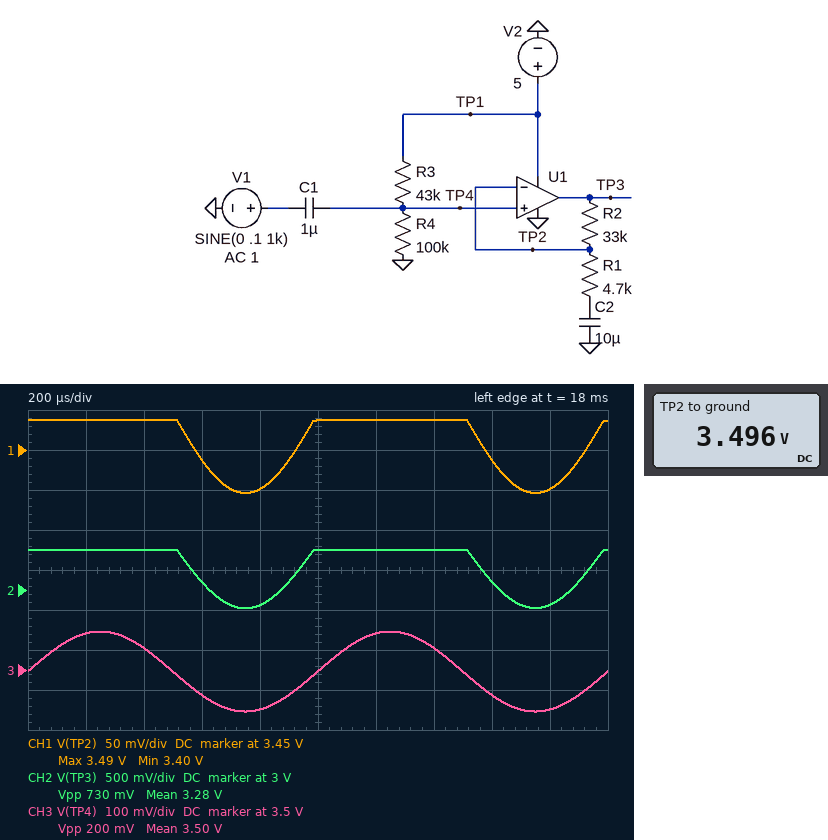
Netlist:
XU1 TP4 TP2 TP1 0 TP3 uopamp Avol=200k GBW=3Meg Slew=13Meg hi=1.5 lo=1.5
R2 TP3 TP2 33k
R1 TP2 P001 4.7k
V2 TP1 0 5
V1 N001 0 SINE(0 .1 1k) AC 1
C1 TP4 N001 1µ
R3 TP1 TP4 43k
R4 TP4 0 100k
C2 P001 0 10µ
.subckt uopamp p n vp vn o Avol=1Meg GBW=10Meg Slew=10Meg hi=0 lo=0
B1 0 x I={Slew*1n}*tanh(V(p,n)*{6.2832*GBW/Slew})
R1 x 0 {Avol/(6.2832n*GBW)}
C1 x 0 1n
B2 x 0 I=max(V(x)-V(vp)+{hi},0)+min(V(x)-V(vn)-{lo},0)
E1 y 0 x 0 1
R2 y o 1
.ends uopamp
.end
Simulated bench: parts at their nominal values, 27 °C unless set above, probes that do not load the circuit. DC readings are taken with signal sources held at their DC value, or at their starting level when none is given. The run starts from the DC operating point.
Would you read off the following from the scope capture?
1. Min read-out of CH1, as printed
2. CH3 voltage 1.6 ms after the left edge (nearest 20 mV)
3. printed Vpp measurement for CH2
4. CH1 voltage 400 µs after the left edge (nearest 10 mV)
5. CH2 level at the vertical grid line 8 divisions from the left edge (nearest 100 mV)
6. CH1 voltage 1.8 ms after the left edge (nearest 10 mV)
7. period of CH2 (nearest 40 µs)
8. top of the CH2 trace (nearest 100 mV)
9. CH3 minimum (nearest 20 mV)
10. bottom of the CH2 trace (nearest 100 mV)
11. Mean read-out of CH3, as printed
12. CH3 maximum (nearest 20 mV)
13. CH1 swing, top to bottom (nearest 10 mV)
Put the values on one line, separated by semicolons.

3.40 V; 3.44 V; 730 mV; 3.49 V; 3.1 V; 3.40 V; 1.00 ms; 3.5 V; 3.40 V; 2.8 V; 3.50 V; 3.60 V; 90 mV
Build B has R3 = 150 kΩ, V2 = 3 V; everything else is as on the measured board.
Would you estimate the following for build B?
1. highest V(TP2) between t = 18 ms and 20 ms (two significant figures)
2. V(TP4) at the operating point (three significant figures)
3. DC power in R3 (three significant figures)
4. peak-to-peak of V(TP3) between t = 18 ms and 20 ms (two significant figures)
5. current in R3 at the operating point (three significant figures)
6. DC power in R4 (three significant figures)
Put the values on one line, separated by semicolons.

1.5 V; 1.20 V; 21.6 µW; 3.1 mV; 12.0 µA; 14.4 µW
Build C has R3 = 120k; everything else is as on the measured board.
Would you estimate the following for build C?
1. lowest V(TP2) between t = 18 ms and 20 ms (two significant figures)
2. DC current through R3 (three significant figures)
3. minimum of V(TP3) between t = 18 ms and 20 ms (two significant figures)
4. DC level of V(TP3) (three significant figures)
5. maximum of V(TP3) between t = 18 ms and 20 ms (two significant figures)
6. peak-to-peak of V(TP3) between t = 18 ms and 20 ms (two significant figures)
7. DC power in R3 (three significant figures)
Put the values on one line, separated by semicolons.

2.2 V; 22.7 µA; 1.5 V; 2.27 V; 3.1 V; 1.6 V; 62.0 µW
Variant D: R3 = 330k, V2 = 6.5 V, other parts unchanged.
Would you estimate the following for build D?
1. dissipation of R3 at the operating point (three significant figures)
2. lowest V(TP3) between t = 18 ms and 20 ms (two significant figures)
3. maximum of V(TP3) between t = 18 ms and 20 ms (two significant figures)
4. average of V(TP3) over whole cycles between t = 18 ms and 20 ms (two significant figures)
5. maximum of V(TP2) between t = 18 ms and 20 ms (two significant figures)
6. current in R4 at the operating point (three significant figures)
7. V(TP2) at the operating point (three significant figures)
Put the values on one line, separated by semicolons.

75.4 µW; 1.5 V; 2.2 V; 1.7 V; 1.6 V; 15.1 µA; 1.51 V
